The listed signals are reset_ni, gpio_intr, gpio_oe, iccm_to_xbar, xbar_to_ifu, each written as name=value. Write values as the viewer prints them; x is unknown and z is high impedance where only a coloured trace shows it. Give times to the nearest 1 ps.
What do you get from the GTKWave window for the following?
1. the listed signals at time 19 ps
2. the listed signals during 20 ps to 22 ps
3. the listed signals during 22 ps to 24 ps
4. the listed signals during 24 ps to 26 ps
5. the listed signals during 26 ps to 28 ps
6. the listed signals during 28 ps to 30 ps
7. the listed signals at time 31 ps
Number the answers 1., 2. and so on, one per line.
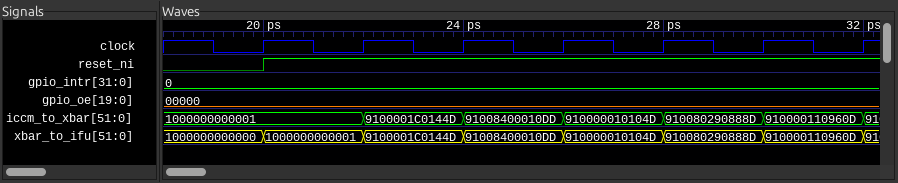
1. reset_ni=0, gpio_intr=0, gpio_oe=00000, iccm_to_xbar=1000000000001, xbar_to_ifu=1000000000000
2. reset_ni=1, gpio_intr=0, gpio_oe=00000, iccm_to_xbar=1000000000001, xbar_to_ifu=1000000000001
3. reset_ni=1, gpio_intr=0, gpio_oe=00000, iccm_to_xbar=9100001C0144D, xbar_to_ifu=9100001C0144D
4. reset_ni=1, gpio_intr=0, gpio_oe=00000, iccm_to_xbar=91008400010DD, xbar_to_ifu=91008400010DD
5. reset_ni=1, gpio_intr=0, gpio_oe=00000, iccm_to_xbar=910000010104D, xbar_to_ifu=910000010104D
6. reset_ni=1, gpio_intr=0, gpio_oe=00000, iccm_to_xbar=910080290888D, xbar_to_ifu=910080290888D
7. reset_ni=1, gpio_intr=0, gpio_oe=00000, iccm_to_xbar=910000110960D, xbar_to_ifu=910000110960D
